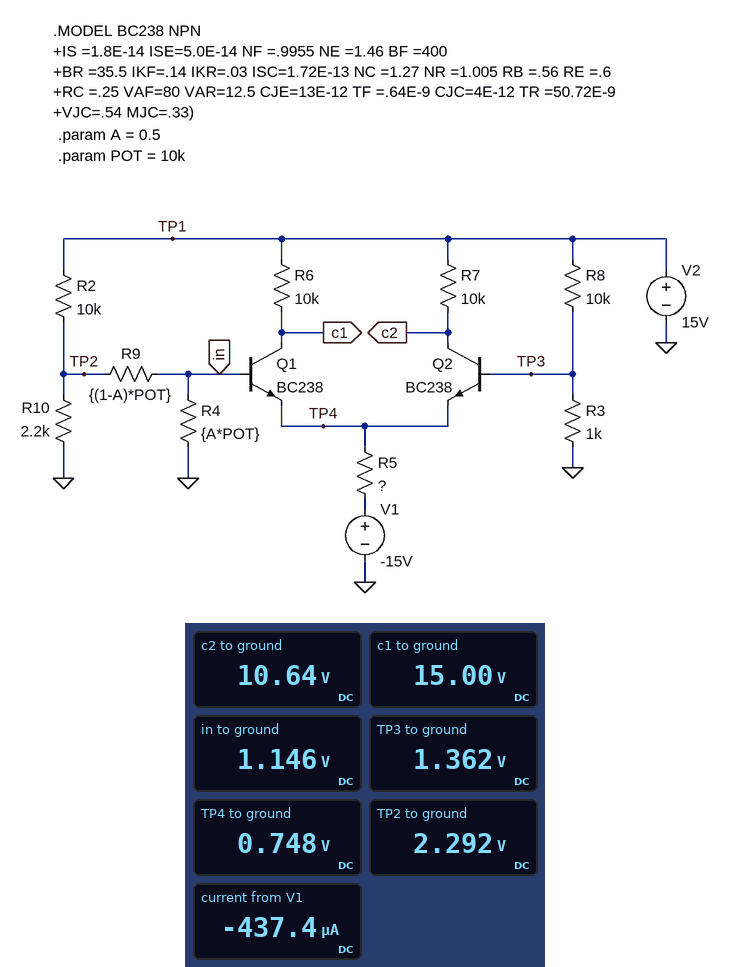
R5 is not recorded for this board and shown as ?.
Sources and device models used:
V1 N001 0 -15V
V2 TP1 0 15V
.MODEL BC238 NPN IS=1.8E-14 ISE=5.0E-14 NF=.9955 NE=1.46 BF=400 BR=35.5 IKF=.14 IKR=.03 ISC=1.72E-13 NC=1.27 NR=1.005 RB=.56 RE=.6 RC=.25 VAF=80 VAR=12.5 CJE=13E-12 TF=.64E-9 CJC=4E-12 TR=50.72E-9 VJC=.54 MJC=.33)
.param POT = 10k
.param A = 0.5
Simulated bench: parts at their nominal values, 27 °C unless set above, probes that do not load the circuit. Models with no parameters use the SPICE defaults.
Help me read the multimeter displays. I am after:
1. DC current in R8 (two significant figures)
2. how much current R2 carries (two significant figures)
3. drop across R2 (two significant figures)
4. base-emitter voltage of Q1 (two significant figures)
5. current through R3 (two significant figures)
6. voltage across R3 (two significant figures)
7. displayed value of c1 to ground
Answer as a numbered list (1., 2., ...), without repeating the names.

1. 1.4 mA
2. 1.3 mA
3. 13 V
4. 400 mV
5. 1.4 mA
6. 1.4 V
7. 15.00 V
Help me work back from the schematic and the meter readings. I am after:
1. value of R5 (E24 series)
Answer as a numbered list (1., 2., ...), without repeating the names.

1. 36 kΩ
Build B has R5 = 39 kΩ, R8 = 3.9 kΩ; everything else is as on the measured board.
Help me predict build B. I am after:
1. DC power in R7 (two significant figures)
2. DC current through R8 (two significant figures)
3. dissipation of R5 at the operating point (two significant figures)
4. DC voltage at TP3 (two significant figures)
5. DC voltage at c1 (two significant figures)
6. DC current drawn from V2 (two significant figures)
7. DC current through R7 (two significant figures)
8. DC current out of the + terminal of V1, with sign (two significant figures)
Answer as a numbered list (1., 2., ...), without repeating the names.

1. 2.0 mW
2. 3.1 mA
3. 7.8 mW
4. 3.1 V
5. 15 V
6. 4.8 mA
7. 450 µA
8. -450 µA
